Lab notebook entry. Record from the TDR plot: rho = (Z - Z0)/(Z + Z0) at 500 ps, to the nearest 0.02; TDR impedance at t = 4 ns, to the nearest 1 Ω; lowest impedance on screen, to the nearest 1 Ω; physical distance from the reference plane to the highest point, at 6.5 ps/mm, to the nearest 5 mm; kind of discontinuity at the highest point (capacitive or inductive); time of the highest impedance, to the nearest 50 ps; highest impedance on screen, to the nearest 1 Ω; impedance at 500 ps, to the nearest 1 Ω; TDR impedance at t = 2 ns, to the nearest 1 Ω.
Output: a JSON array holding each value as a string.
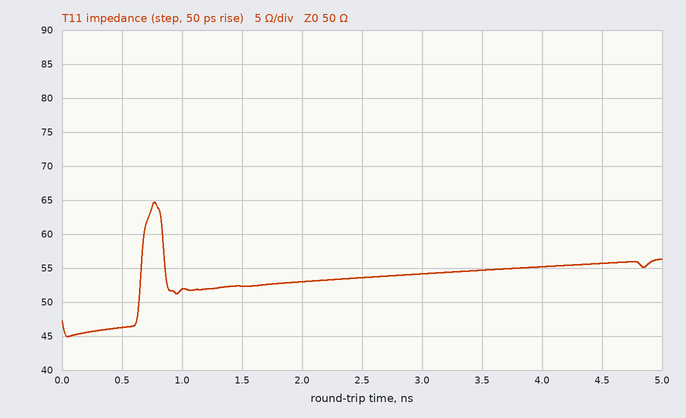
["-0.04", "55 Ω", "45 Ω", "60 mm", "inductive", "750 ps", "65 Ω", "46 Ω", "53 Ω"]
